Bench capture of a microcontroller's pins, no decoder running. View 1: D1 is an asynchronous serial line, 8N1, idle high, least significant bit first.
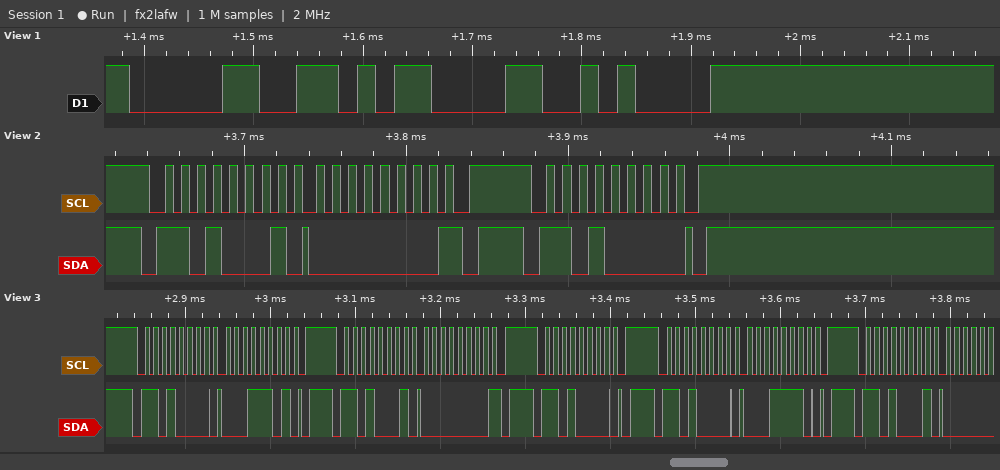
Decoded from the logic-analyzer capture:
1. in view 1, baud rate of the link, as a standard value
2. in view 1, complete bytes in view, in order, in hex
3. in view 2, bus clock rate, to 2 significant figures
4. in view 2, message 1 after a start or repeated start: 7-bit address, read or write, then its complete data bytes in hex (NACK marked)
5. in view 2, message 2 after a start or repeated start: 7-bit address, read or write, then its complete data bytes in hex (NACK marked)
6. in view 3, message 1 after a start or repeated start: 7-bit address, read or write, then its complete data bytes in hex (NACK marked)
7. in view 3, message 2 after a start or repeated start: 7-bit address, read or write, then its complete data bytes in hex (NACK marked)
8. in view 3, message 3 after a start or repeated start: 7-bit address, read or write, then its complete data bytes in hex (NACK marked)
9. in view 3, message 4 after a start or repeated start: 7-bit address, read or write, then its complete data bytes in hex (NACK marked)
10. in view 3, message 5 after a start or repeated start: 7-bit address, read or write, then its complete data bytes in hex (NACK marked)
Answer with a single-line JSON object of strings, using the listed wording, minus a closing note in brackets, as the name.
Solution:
{"in view 1, baud rate of the link, as a standard value": "57600 baud", "in view 1, complete bytes in view, in order, in hex": "30 0D 0A", "in view 2, bus clock rate, to 2 significant figures": "100 kHz", "in view 2, message 1 after a start or repeated start: 7-bit address, read or write, then its complete data bytes in hex": "0x68 read: 00 NACK", "in view 2, message 2 after a start or repeated start: 7-bit address, read or write, then its complete data bytes in hex": "0x68 write", "in view 3, message 1 after a start or repeated start: 7-bit address, read or write, then its complete data bytes in hex": "0x68 write: 1D", "in view 3, message 2 after a start or repeated start: 7-bit address, read or write, then its complete data bytes in hex": "0x68 read: 00 NACK", "in view 3, message 3 after a start or repeated start: 7-bit address, read or write, then its complete data bytes in hex": "0x68 write", "in view 3, message 4 after a start or repeated start: 7-bit address, read or write, then its complete data bytes in hex": "0x68 write: 1E", "in view 3, message 5 after a start or repeated start: 7-bit address, read or write, then its complete data bytes in hex": "0x68 read"}
